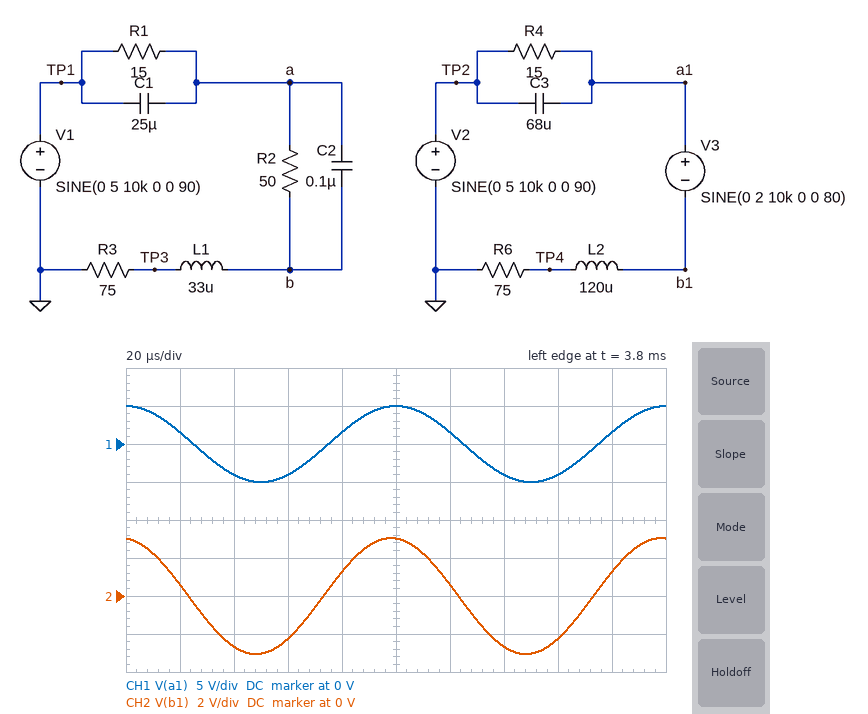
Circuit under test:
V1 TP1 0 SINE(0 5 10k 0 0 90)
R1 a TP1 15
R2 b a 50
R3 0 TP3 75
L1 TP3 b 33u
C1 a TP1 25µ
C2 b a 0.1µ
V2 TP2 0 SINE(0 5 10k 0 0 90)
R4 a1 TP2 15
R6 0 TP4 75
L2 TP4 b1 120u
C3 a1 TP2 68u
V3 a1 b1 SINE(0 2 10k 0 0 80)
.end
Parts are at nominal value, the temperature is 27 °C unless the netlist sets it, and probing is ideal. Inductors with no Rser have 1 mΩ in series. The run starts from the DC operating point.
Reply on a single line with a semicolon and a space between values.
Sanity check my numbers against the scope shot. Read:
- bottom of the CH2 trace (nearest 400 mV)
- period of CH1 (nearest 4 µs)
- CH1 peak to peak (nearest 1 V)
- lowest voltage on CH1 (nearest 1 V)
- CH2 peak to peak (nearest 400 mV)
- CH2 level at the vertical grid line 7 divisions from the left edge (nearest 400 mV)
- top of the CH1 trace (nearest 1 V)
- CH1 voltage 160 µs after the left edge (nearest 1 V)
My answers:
-3.2 V; 100 µs; 10 V; -5 V; 6.0 V; -2.8 V; 5 V; -4 V
